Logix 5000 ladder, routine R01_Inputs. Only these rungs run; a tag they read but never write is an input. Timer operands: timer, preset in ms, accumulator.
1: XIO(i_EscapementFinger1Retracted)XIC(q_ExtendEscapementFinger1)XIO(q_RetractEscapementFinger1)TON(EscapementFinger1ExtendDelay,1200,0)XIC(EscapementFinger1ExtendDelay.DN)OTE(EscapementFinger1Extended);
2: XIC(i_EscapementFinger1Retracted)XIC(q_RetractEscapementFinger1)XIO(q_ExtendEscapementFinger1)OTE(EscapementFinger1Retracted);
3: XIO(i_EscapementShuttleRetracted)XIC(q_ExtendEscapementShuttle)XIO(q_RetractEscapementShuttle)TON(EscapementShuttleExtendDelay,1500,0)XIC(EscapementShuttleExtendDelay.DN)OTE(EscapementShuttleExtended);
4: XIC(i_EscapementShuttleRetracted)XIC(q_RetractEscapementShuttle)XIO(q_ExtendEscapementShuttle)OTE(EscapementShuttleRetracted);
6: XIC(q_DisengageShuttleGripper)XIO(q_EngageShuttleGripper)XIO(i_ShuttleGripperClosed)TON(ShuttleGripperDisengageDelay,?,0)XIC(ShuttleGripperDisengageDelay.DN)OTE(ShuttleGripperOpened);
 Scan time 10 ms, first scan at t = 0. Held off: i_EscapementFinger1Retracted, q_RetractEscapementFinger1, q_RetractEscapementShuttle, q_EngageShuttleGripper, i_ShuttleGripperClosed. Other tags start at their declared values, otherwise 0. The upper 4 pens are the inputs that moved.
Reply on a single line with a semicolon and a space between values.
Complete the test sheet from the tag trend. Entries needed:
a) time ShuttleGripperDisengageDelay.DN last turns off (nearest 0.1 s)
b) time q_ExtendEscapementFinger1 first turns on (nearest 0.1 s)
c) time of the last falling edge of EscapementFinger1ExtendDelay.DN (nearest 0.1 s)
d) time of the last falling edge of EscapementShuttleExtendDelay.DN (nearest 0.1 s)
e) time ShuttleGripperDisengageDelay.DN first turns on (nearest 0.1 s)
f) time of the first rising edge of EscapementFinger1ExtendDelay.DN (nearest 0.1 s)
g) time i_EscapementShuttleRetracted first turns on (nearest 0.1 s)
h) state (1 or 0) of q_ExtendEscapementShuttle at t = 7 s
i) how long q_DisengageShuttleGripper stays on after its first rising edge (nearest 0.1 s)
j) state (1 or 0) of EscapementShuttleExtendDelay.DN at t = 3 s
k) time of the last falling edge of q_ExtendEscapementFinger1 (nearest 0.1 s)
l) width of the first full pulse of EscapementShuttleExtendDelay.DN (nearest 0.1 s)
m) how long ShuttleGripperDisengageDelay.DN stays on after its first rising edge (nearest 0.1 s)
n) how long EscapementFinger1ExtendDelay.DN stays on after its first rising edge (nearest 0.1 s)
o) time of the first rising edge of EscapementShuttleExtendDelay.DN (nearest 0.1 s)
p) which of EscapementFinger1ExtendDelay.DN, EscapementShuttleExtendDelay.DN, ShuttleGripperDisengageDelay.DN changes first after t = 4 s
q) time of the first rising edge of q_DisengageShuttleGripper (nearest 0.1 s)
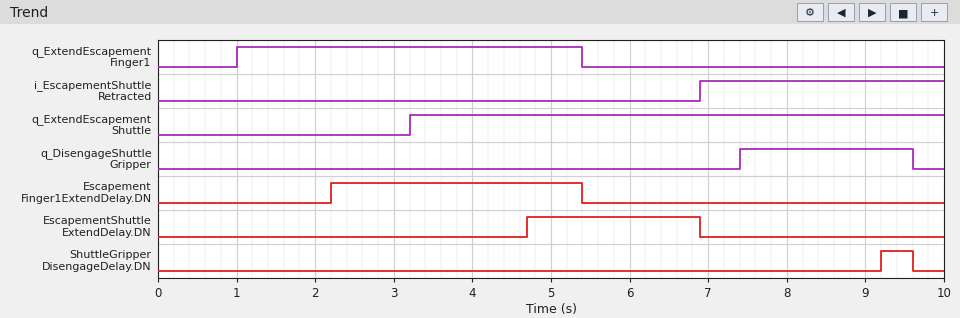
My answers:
9.6 s; 1.0 s; 5.4 s; 6.9 s; 9.2 s; 2.2 s; 6.9 s; 1; 2.2 s; 0; 5.4 s; 2.2 s; 0.4 s; 3.2 s; 4.7 s; EscapementShuttleExtendDelay.DN; 7.4 s
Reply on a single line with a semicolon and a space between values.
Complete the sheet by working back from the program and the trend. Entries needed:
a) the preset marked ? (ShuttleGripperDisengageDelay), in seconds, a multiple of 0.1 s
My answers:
1.8 s
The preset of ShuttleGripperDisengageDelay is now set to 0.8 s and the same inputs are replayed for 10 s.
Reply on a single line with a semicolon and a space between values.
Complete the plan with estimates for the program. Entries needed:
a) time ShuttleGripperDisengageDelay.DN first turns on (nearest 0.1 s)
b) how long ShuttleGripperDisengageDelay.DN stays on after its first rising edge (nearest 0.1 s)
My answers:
8.2 s; 1.4 s
